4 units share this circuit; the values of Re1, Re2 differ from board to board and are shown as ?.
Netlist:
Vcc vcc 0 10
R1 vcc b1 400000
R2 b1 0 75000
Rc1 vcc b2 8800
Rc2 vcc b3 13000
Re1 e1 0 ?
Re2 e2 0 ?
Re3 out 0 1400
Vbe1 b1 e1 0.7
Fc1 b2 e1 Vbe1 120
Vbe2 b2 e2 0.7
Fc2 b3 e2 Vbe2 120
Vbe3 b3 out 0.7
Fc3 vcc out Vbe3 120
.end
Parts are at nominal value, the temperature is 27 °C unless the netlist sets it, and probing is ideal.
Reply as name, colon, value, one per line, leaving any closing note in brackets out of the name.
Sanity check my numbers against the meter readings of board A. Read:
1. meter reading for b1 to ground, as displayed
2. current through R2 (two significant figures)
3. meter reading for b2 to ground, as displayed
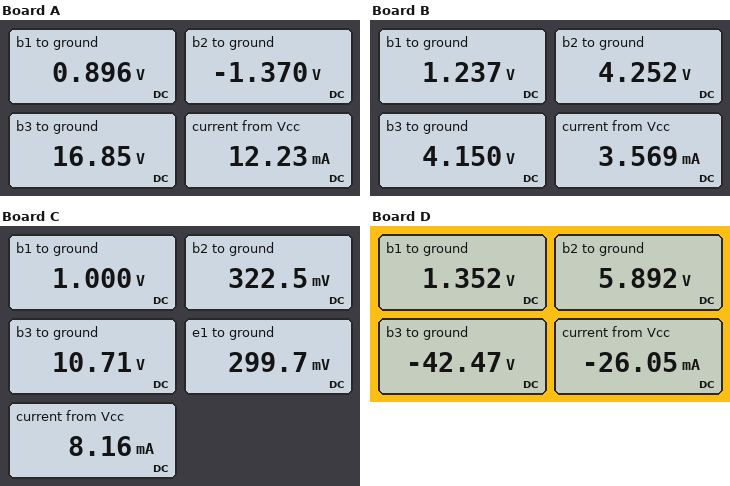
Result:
meter reading for b1 to ground, as displayed: 0.896 V
current through R2: 12 µA
meter reading for b2 to ground, as displayed: -1.370 V
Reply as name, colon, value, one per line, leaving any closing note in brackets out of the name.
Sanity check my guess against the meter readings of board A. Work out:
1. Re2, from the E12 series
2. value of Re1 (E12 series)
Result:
Re2, from the E12 series: 3.3 kΩ
value of Re1: 150 Ω
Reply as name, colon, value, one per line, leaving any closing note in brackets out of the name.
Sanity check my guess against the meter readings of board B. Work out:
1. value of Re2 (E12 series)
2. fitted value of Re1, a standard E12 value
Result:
value of Re2: 8.2 kΩ
fitted value of Re1, a standard E12 value: 820 Ω
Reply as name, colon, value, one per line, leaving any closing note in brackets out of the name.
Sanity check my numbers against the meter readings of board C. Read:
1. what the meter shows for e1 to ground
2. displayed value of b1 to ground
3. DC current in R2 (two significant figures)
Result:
what the meter shows for e1 to ground: 299.7 mV
displayed value of b1 to ground: 1.000 V
DC current in R2: 13 µA
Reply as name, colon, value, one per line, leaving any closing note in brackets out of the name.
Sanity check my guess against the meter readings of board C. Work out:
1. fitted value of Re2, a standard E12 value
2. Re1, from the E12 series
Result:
fitted value of Re2, a standard E12 value: 3.3 kΩ
Re1, from the E12 series: 270 Ω
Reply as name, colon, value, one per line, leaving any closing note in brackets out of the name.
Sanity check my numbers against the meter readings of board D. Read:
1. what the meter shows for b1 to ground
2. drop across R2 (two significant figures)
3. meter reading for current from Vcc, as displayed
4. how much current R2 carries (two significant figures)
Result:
what the meter shows for b1 to ground: 1.352 V
drop across R2: 1.4 V
meter reading for current from Vcc, as displayed: -26.05 mA
how much current R2 carries: 18 µA
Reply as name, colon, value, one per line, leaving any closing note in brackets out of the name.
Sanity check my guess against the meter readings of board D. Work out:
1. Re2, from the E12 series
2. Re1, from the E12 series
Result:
Re2, from the E12 series: 1.2 kΩ
Re1, from the E12 series: 1.5 kΩ
